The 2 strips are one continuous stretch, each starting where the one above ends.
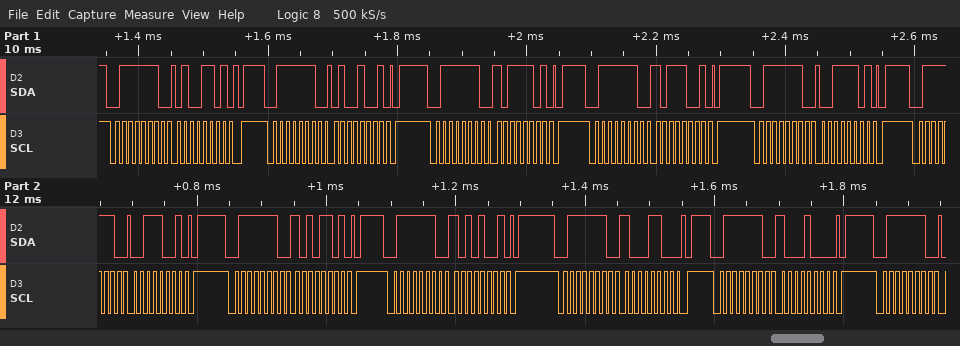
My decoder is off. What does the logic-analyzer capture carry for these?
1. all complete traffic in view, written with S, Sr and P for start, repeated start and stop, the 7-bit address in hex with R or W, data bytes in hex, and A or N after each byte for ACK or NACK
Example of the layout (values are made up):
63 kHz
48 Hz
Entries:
S 3FW A 4D A P S 3FW A 49 A P S 3FW A BD A P S 3FW A B9 A P S 3FW A 3D A P S 3FW A 39 A P S 3FW A AD A P S 3FW A A9 A P S 3FW A 8C A P S 3FW A 88 A P S 3FW A
